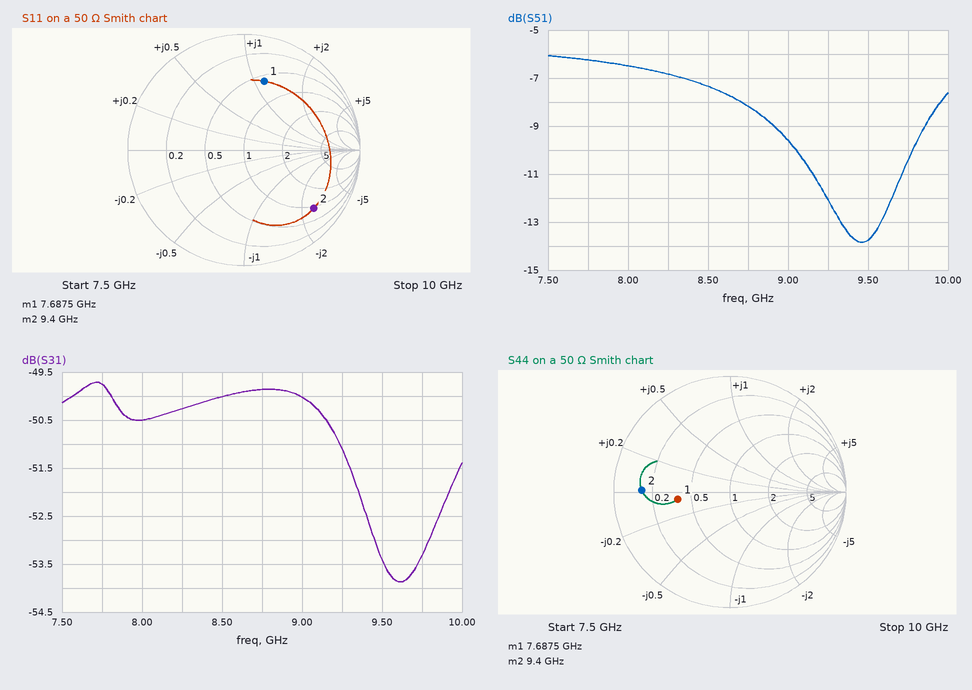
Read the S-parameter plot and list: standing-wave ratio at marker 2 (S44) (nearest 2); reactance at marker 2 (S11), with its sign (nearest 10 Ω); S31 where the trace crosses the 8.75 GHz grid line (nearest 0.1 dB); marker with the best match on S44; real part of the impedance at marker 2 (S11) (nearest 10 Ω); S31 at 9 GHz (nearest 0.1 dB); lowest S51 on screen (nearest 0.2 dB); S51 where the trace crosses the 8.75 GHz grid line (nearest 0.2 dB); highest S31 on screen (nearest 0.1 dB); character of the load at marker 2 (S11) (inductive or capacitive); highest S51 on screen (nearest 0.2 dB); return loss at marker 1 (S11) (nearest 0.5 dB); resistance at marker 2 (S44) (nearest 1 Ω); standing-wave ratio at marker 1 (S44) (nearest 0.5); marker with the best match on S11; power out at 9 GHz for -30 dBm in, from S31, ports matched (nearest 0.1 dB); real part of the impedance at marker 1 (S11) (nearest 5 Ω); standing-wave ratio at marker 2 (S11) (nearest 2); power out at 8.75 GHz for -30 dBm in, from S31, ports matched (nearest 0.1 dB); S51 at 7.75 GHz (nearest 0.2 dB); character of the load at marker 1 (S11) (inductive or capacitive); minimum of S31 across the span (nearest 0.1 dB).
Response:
8
-120 Ω
-49.9 dB
marker 1
50 Ω
-50.0 dB
-13.8 dB
-8.2 dB
-49.7 dB
capacitive
-6.0 dB
4.0 dB
7 Ω
2.5
marker 1
-80.0 dBm
30 Ω
8
-79.9 dBm
-6.2 dB
inductive
-53.9 dB
